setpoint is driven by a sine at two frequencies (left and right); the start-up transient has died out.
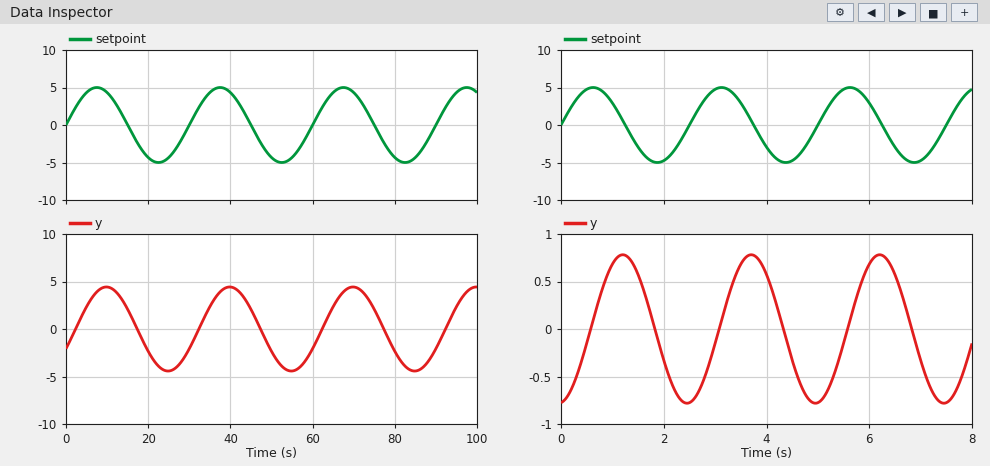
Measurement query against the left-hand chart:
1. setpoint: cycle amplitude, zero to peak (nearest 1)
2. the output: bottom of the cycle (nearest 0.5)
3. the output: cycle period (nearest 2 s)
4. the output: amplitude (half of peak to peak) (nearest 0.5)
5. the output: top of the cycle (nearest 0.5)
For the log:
5
-4.5
30 s
4.5
4.5
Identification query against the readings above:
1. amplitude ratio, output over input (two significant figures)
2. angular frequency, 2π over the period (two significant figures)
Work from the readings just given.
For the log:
0.90
0.21 rad/s
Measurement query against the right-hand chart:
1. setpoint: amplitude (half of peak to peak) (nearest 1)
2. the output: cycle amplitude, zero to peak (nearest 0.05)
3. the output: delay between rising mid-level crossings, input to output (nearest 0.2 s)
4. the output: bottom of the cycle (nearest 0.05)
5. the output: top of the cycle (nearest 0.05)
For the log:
5
0.80
0.6 s
-0.80
0.80
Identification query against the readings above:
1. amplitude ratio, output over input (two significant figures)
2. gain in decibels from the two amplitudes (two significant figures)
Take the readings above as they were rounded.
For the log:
0.16
-16 dB
